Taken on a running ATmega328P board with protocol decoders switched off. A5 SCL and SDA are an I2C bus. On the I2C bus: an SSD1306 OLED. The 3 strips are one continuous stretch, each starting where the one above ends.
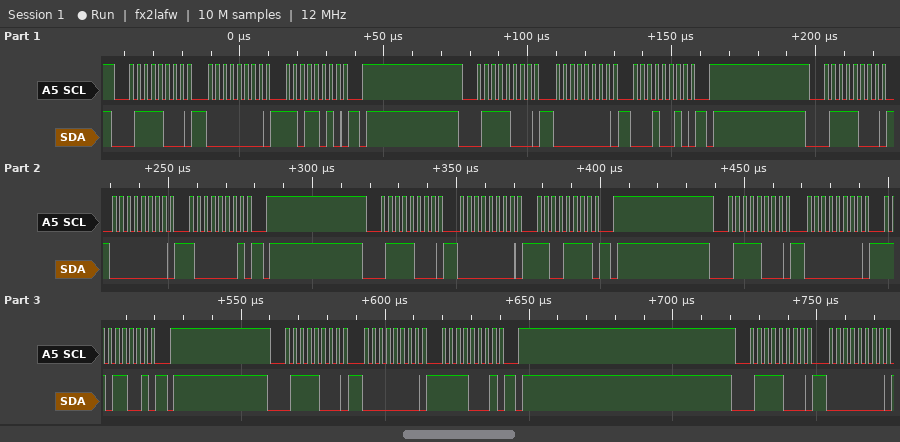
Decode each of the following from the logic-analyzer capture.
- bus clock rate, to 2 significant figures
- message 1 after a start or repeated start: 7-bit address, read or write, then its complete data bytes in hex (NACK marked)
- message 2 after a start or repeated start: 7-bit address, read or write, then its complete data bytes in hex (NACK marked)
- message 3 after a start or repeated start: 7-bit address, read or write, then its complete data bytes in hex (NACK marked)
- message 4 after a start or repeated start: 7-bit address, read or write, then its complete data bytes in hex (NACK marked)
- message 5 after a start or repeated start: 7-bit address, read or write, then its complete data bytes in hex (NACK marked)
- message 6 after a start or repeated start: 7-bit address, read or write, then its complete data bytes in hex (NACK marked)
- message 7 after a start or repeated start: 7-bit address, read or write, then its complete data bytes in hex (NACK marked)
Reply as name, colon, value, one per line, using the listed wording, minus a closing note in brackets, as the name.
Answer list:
bus clock rate, to 2 significant figures: 400 kHz
message 1 after a start or repeated start: 7-bit address, read or write, then its complete data bytes in hex: 0x3C write: 00 DA
message 2 after a start or repeated start: 7-bit address, read or write, then its complete data bytes in hex: 0x3C write: 00 12
message 3 after a start or repeated start: 7-bit address, read or write, then its complete data bytes in hex: 0x3C write: 00 81
message 4 after a start or repeated start: 7-bit address, read or write, then its complete data bytes in hex: 0x3C write: 00 CF
message 5 after a start or repeated start: 7-bit address, read or write, then its complete data bytes in hex: 0x3C write: 00 D9
message 6 after a start or repeated start: 7-bit address, read or write, then its complete data bytes in hex: 0x3C write: 00 F1
message 7 after a start or repeated start: 7-bit address, read or write, then its complete data bytes in hex: 0x3C write: 00
